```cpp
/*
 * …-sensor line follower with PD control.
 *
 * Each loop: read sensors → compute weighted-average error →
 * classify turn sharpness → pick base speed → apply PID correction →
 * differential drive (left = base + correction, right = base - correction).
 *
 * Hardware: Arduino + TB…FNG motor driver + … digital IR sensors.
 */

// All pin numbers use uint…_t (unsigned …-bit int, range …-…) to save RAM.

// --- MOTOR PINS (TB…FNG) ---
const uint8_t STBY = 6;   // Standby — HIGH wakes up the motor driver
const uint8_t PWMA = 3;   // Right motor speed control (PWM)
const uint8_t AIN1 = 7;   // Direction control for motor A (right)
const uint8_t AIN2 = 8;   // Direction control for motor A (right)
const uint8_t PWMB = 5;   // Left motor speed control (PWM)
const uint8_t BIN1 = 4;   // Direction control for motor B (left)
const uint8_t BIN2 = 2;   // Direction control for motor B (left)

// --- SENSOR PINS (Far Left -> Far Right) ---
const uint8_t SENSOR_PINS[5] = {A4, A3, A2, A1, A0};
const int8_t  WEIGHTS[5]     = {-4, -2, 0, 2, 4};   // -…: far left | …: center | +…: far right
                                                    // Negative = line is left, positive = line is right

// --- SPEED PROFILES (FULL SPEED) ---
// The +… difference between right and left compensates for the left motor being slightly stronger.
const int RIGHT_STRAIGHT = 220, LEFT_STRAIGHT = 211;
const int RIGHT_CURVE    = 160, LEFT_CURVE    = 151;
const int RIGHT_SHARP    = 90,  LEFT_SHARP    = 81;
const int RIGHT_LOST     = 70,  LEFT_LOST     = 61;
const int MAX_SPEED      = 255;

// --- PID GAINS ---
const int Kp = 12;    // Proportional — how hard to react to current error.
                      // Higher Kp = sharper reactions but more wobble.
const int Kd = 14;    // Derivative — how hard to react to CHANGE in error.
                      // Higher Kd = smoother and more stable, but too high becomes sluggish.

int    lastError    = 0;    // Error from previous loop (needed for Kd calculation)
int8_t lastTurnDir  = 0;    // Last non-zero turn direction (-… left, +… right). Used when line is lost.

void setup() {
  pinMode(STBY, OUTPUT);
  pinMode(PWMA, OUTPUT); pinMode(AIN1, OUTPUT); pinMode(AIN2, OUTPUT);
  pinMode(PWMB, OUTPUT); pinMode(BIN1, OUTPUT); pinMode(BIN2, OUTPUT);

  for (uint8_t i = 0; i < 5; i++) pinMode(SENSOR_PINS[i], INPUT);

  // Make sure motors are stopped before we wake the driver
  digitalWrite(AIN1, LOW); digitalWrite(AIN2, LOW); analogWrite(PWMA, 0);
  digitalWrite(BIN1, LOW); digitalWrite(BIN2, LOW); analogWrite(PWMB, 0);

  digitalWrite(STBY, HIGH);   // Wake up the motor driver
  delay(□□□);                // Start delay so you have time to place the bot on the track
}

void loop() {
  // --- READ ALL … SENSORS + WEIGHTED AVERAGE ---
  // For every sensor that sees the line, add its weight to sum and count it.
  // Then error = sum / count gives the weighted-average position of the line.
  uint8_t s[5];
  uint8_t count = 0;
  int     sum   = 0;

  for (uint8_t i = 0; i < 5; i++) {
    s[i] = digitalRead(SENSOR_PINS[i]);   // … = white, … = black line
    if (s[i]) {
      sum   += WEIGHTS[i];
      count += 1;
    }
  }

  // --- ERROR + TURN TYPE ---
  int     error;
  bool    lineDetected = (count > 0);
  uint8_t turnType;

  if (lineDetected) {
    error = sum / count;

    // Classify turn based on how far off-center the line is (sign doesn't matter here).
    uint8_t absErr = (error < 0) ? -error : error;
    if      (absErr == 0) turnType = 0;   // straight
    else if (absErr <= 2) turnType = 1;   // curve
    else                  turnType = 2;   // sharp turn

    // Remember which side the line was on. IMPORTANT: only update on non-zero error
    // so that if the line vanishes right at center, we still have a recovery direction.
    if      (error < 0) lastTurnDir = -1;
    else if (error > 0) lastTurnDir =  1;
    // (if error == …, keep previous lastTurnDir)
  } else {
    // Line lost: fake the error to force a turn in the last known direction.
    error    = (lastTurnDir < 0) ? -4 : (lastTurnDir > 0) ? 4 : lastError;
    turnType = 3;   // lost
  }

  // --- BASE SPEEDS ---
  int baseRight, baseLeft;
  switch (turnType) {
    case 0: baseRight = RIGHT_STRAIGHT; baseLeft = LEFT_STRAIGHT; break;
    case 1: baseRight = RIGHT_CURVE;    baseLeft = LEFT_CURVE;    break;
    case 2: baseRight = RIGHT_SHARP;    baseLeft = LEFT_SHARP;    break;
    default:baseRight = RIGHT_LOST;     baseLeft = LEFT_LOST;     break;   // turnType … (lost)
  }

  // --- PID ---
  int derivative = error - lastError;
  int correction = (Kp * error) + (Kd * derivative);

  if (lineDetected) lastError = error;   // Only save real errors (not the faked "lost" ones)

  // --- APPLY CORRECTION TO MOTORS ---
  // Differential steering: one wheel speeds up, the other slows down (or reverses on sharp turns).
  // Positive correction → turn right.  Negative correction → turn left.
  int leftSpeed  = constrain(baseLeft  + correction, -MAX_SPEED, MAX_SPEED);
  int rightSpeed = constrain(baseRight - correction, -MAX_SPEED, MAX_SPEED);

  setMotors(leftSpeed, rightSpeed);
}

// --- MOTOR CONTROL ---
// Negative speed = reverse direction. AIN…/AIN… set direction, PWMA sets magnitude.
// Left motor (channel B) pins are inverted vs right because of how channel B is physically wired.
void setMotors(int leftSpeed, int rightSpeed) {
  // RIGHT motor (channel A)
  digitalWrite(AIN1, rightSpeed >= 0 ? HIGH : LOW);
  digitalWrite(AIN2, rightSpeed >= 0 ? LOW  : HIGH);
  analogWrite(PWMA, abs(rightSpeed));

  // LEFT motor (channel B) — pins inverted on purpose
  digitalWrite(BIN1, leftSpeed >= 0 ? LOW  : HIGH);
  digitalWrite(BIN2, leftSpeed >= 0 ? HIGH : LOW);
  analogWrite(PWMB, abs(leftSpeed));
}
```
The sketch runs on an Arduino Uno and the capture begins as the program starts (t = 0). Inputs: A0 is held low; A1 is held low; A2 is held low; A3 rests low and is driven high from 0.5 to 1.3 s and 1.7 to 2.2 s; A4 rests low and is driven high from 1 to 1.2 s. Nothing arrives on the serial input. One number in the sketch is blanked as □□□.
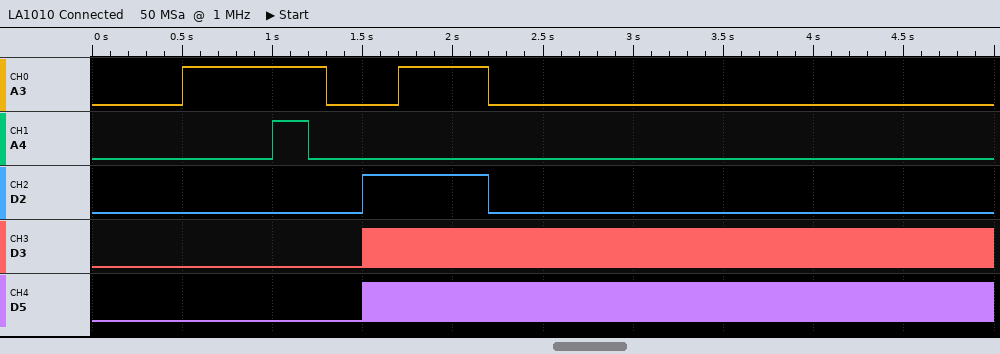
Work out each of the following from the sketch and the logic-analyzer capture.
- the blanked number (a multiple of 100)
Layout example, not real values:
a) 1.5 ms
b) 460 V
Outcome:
a) 1500
